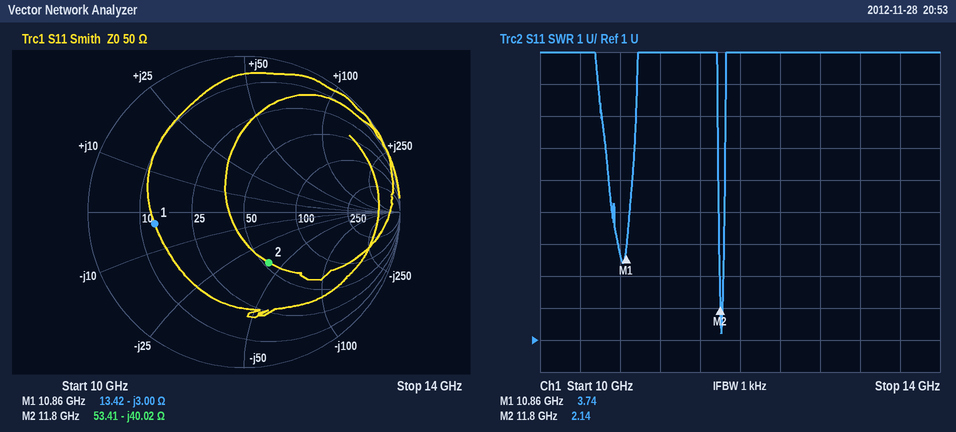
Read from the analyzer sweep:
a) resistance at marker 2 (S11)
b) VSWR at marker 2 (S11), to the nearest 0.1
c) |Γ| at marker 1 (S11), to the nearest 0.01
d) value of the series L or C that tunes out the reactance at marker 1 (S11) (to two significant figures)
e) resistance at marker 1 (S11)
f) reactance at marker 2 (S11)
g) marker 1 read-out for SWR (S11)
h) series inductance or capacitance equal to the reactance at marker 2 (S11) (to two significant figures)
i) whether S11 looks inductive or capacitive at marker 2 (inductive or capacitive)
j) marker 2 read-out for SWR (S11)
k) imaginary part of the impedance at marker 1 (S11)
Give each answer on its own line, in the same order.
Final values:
53.41 Ω
2.1
0.58
44 pH
13.42 Ω
-40.02 Ω
3.74
340 fF
capacitive
2.14
-3.00 Ω
